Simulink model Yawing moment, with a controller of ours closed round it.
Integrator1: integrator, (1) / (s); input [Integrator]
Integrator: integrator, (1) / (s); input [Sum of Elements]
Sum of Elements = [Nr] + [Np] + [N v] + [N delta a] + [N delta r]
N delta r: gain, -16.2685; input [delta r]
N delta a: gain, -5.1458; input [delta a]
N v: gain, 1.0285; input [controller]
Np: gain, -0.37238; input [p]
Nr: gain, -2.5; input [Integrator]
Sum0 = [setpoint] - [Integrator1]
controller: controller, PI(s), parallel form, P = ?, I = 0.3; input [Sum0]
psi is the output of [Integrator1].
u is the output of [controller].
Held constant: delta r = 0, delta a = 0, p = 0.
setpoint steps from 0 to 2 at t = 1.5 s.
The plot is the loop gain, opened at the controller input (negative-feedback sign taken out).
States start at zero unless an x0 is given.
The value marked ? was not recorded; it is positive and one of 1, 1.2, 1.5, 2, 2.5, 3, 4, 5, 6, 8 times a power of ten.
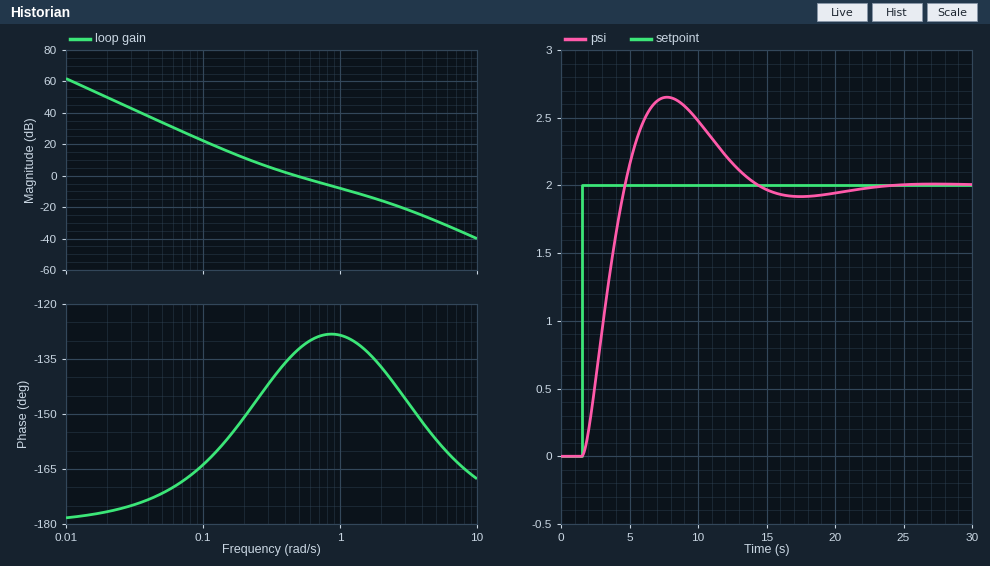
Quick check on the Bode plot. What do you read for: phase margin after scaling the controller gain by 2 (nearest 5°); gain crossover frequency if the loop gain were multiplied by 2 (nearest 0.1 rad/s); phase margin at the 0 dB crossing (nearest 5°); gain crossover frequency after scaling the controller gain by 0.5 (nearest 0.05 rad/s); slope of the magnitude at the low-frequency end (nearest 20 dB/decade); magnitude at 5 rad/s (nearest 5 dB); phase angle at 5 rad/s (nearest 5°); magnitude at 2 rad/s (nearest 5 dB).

50°
0.8 rad/s
45°
0.30 rad/s
-40 dB/decade
-30 dB
-155°
-15 dB
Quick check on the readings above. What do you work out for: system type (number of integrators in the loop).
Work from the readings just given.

2
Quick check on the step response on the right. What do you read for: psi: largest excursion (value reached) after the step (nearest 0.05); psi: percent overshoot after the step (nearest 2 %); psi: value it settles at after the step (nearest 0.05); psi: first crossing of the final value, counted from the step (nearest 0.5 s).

2.65
32 %
2.00
3.0 s
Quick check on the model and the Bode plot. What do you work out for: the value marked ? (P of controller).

1
